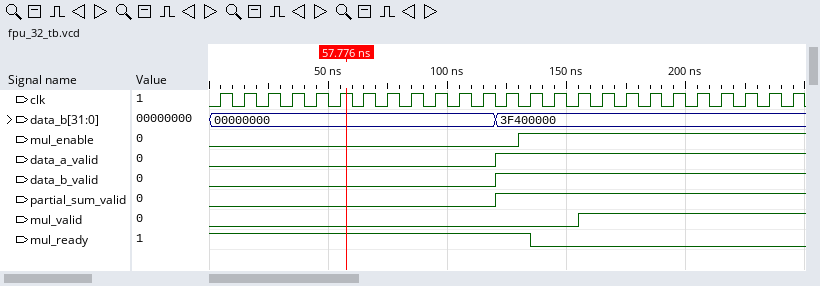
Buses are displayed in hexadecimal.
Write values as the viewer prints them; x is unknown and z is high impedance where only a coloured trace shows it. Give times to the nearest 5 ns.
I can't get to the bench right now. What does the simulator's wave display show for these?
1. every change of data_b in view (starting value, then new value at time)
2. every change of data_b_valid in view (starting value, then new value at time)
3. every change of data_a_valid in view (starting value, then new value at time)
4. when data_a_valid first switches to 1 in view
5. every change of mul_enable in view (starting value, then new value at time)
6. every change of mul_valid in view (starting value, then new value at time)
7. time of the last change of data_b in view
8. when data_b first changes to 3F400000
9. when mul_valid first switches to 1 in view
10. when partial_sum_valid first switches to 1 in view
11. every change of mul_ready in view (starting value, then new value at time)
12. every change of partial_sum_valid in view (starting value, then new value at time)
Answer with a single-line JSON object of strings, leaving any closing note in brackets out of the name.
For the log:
{"every change of data_b in view": "00000000, 3F400000 at 120 ns", "every change of data_b_valid in view": "0, 1 at 120 ns", "every change of data_a_valid in view": "0, 1 at 120 ns", "when data_a_valid first switches to 1 in view": "120 ns", "every change of mul_enable in view": "0, 1 at 130 ns", "every change of mul_valid in view": "0, 1 at 155 ns", "time of the last change of data_b in view": "120 ns", "when data_b first changes to 3F400000": "120 ns", "when mul_valid first switches to 1 in view": "155 ns", "when partial_sum_valid first switches to 1 in view": "120 ns", "every change of mul_ready in view": "1, 0 at 135 ns", "every change of partial_sum_valid in view": "0, 1 at 120 ns"}
